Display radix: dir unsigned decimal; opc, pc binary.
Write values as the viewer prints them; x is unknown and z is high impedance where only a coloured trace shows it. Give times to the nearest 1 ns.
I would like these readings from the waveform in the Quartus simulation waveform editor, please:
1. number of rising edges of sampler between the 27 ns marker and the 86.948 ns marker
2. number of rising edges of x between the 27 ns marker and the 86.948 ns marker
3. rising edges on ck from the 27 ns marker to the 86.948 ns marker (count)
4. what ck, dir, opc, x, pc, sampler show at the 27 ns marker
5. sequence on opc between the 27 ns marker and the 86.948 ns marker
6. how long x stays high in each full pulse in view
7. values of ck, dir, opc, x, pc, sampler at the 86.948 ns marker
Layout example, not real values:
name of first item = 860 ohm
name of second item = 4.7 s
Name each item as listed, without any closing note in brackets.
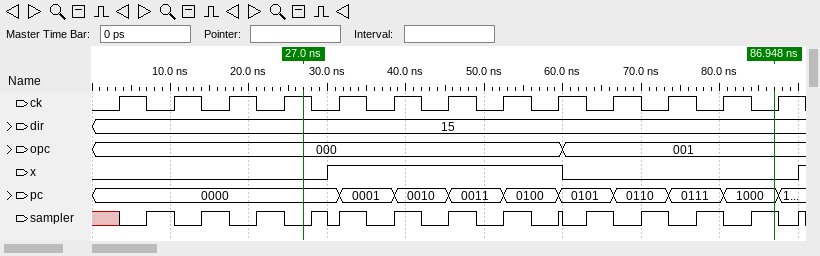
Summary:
number of rising edges of sampler between the 27 ns marker and the 86.948 ns marker = 10
number of rising edges of x between the 27 ns marker and the 86.948 ns marker = 1
rising edges on ck from the 27 ns marker to the 86.948 ns marker = 8
what ck, dir, opc, x, pc, sampler show at the 27 ns marker = ck=1, dir=15, opc=000, x=0, pc=0000, sampler=0
sequence on opc between the 27 ns marker and the 86.948 ns marker = 000, 001
how long x stays high in each full pulse in view = 30 ns
values of ck, dir, opc, x, pc, sampler at the 86.948 ns marker = ck=0, dir=15, opc=001, x=0, pc=1000, sampler=1
